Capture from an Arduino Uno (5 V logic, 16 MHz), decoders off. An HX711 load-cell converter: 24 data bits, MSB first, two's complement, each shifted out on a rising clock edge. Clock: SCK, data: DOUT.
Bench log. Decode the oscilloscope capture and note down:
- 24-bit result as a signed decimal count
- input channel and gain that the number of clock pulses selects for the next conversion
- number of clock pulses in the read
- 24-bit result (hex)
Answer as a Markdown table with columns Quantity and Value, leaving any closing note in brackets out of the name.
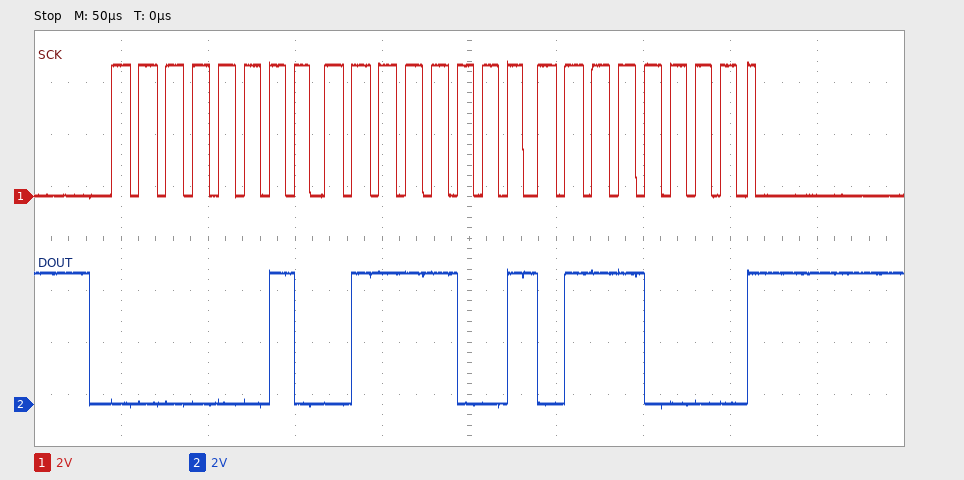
| Quantity | Value |
|---|---|
| 24-bit result as a signed decimal count | 162160 |
| input channel and gain that the number of clock pulses selects for the next conversion | channel A, gain 128 |
| number of clock pulses in the read | 25 |
| 24-bit result | 0x027970 |
